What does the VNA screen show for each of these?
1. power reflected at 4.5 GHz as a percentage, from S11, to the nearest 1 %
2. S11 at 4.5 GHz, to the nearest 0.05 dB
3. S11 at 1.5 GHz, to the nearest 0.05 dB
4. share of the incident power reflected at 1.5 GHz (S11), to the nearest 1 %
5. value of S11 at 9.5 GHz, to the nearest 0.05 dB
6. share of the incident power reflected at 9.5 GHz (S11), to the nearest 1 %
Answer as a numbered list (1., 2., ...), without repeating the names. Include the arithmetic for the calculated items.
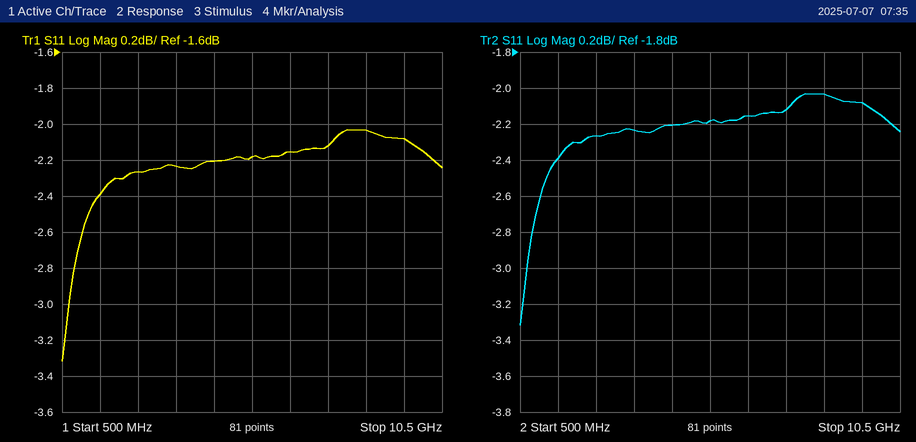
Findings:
1. 10^(-2.2/10) ≈ 60 %
2. -2.20 dB
3. -2.40 dB
4. 10^(-2.4/10) ≈ 58 %
5. -2.10 dB
6. 10^(-2.1/10) ≈ 62 %
